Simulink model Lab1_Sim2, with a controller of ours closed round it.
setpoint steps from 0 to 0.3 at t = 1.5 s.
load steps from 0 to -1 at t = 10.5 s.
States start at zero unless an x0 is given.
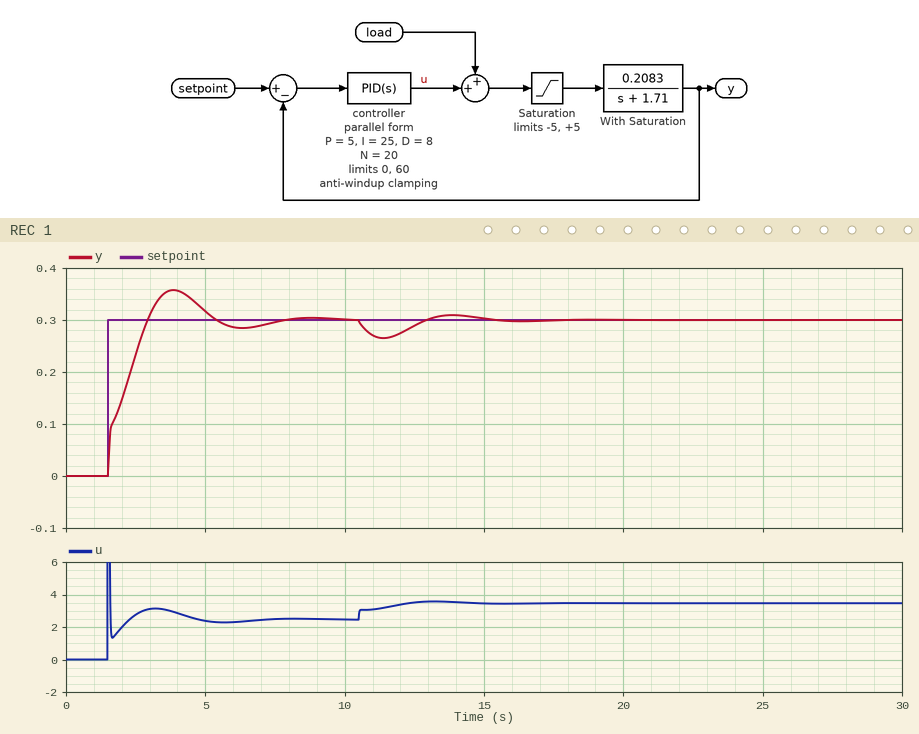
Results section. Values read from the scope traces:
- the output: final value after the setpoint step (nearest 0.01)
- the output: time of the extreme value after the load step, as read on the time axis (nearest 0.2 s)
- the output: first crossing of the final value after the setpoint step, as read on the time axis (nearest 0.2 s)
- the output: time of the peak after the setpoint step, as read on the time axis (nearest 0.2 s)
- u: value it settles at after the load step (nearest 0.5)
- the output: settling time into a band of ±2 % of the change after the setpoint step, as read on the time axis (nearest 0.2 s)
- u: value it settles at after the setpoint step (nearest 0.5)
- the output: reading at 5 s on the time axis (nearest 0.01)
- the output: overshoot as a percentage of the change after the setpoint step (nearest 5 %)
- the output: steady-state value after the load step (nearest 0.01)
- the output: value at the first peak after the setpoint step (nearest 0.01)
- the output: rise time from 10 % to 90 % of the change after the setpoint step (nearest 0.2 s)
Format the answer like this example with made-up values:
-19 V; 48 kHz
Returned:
0.30; 11.4 s; 3.0 s; 3.8 s; 3.5; 7.4 s; 2.5; 0.32; 20 %; 0.30; 0.36; 1.2 s
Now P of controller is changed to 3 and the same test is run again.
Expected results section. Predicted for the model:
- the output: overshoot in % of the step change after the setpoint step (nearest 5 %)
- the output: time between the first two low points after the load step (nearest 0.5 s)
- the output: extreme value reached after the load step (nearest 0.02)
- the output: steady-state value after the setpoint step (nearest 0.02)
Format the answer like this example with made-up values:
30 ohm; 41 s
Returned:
25 %; 5.0 s; 0.26; 0.30
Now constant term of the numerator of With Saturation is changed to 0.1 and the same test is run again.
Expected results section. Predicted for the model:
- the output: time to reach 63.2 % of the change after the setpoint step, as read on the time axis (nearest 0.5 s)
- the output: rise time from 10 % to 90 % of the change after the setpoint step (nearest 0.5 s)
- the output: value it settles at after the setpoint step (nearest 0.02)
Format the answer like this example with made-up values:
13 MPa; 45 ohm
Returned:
2.5 s; 2.0 s; 0.30
